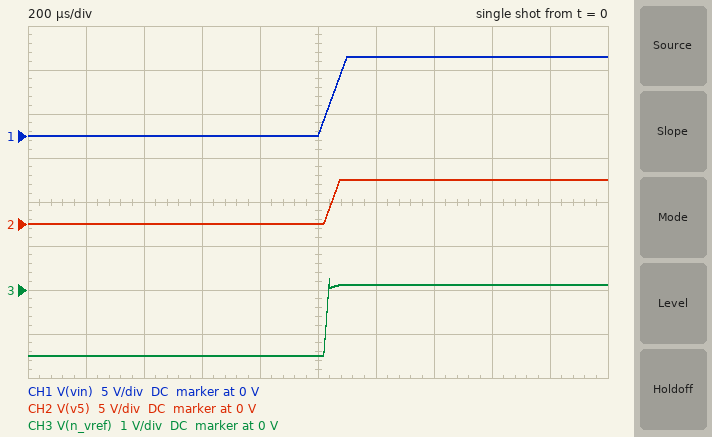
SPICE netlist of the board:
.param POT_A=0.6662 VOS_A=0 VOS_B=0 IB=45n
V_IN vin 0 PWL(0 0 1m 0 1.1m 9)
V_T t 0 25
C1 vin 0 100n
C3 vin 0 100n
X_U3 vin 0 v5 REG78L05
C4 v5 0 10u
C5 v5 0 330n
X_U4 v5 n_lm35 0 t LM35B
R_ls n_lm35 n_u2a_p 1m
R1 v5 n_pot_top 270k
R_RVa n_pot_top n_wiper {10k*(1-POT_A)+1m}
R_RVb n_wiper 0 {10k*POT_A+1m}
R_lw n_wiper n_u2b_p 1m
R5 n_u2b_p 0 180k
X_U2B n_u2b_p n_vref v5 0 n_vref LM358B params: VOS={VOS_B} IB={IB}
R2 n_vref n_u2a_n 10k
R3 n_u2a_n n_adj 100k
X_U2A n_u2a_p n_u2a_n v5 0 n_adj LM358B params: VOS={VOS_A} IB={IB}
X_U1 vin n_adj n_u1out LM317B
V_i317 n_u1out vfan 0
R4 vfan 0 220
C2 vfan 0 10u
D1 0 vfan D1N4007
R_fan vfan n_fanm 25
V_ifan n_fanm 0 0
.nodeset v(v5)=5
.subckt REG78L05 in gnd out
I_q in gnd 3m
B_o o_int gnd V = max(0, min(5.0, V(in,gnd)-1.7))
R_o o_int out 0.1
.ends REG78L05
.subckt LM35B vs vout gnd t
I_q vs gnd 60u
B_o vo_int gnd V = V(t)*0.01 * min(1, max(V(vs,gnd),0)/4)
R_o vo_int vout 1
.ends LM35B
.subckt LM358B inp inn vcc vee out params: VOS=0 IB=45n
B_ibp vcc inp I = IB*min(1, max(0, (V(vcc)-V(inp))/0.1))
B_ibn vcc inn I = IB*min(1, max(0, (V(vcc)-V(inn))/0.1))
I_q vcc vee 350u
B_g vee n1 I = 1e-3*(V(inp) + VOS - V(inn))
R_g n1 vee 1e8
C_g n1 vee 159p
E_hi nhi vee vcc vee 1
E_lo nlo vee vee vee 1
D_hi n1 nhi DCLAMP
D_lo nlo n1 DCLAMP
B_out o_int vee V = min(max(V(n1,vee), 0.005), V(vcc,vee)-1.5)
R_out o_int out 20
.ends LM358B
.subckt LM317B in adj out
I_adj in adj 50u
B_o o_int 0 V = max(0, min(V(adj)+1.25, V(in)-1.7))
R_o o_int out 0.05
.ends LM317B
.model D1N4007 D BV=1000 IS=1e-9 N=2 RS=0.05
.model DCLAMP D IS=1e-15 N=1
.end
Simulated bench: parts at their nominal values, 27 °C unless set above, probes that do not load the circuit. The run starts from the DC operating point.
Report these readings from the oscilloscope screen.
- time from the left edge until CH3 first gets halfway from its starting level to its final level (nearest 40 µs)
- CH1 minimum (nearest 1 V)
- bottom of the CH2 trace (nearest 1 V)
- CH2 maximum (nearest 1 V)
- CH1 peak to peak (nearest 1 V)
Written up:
1.04 ms
0 V
0 V
5 V
9 V
